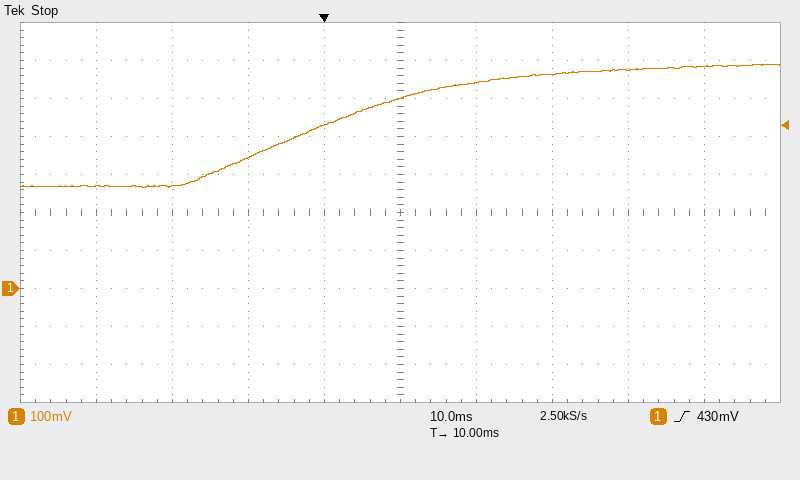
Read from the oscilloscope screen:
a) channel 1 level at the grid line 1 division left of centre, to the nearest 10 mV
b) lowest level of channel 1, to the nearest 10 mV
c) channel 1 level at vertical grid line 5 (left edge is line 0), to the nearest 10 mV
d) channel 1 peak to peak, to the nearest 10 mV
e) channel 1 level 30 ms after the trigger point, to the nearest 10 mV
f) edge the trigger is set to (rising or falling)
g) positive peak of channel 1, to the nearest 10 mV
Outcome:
430 mV
270 mV
500 mV
320 mV
560 mV
rising
590 mV
